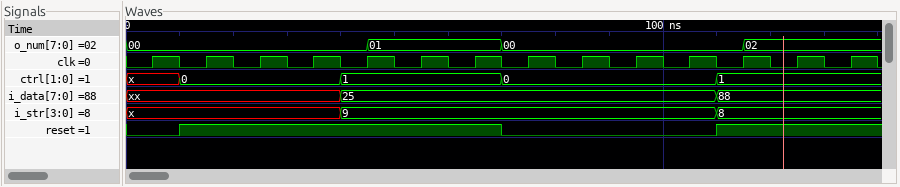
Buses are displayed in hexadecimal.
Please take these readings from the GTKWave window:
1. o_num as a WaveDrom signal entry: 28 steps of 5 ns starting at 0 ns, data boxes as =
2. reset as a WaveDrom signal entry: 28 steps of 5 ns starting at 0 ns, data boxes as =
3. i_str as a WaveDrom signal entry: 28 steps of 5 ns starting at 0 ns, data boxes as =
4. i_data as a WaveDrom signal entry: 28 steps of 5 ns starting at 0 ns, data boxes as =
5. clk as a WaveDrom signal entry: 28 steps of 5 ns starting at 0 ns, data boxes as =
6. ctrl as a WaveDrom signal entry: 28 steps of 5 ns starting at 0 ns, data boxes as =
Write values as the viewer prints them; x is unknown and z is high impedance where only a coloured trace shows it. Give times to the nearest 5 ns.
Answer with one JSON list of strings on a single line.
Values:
["{name: 'o_num', wave: '=........=....=........=....', data: '00 01 00 02'}", "{name: 'reset', wave: '0.1...........0.......1.....'}", "{name: 'i_str', wave: 'x.......=.............=.....', data: '9 8'}", "{name: 'i_data', wave: 'x.......=.............=.....', data: '25 88'}", "{name: 'clk', wave: '0101010101010101010101010101'}", "{name: 'ctrl', wave: 'x.=.....=.....=.......=.....', data: '0 1 0 1'}"]
